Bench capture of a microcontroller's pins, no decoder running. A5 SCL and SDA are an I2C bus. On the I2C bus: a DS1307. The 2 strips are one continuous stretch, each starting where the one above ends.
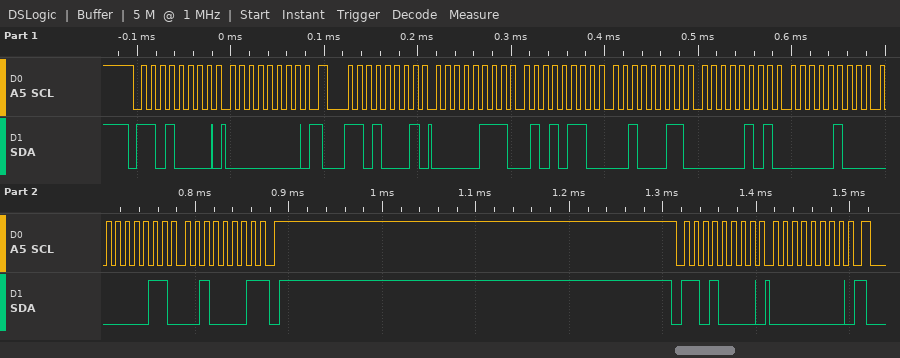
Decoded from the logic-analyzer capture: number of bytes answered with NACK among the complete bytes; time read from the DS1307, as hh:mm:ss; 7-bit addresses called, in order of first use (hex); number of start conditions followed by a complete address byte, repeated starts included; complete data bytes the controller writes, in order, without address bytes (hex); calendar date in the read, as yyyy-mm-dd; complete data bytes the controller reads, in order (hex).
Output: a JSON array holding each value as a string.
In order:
["1", "23:56:07", "0x68", "3", "00 00", "2021-03-04", "07 56 23 05 04 03 21"]
